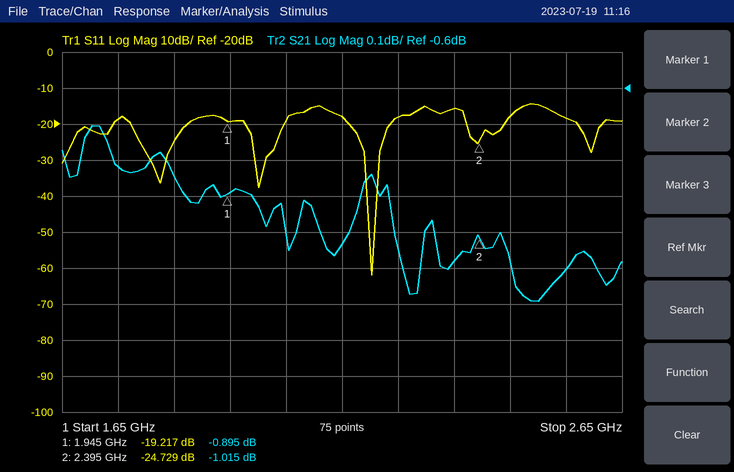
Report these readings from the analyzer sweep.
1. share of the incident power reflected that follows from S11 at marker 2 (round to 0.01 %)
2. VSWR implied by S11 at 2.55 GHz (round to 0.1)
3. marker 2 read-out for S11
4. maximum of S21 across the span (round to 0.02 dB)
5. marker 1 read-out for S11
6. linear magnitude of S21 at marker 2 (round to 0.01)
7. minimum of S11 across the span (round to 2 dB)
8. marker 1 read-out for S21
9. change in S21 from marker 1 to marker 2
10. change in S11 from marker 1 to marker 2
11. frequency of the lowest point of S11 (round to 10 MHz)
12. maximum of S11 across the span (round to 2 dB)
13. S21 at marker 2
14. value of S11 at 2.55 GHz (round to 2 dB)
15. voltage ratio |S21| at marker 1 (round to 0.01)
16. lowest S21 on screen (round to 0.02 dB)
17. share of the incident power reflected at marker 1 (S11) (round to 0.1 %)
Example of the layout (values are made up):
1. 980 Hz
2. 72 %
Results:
1. 0.34 %
2. 1.3
3. -24.729 dB
4. -0.70 dB
5. -19.217 dB
6. 0.89
7. -62 dB
8. -0.895 dB
9. -0.120 dB
10. -5.512 dB
11. 2.20 GHz
12. -14 dB
13. -1.015 dB
14. -18 dB
15. 0.90
16. -1.20 dB
17. 1.2 %
